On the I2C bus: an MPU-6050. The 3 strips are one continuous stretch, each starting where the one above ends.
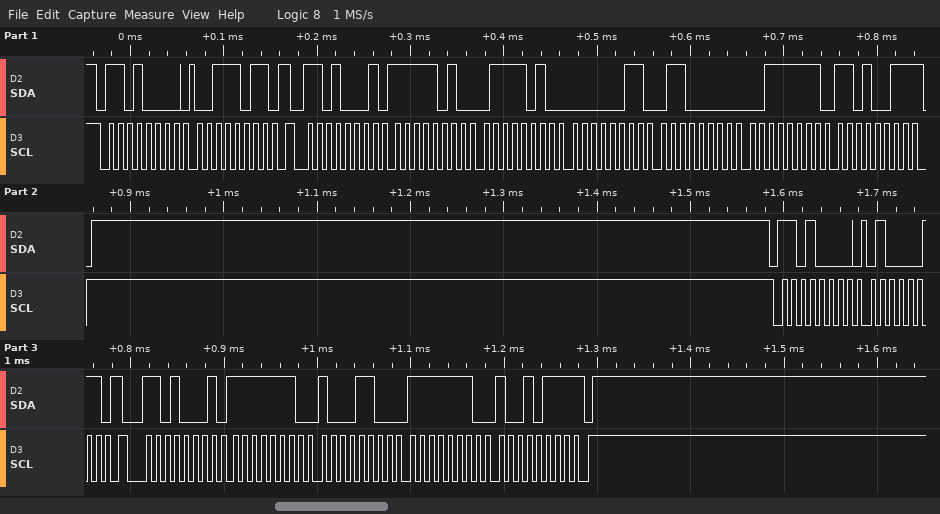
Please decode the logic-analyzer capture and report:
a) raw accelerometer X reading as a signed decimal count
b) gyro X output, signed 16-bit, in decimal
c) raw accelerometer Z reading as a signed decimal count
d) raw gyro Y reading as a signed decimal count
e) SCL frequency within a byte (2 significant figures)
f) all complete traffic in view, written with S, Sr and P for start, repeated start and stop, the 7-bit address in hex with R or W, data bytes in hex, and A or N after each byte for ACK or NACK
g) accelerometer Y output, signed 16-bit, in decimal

-1414
-372
16339
-361
100 kHz
S 68W A 3B A Sr 68R A FA A 7A A 03 A 60 A 3F A D3 N P S 68W A 43 A Sr 68R A FE A 8C A FE A 97 N P
864
